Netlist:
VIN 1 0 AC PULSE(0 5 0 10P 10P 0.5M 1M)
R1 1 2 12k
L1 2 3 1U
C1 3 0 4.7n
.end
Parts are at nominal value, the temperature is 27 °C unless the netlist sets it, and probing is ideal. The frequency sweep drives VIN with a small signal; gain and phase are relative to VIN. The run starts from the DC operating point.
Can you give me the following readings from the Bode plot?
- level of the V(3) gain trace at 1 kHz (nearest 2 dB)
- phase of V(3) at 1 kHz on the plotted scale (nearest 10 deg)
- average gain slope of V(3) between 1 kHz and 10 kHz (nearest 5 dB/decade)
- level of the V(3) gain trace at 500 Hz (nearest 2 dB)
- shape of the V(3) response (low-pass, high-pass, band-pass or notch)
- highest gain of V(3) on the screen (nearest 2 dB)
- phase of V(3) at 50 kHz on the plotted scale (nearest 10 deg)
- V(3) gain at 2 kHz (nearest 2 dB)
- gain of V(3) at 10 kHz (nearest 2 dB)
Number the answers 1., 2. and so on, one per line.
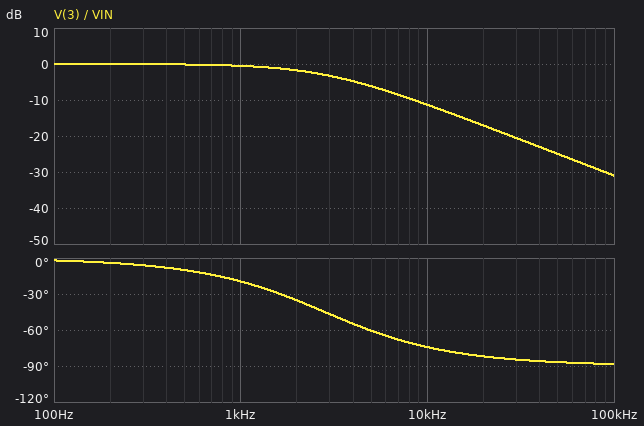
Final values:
1. 0 dB
2. -20 deg
3. -10 dB/decade
4. 0 dB
5. low-pass
6. 0 dB
7. -90 deg
8. -2 dB
9. -12 dB
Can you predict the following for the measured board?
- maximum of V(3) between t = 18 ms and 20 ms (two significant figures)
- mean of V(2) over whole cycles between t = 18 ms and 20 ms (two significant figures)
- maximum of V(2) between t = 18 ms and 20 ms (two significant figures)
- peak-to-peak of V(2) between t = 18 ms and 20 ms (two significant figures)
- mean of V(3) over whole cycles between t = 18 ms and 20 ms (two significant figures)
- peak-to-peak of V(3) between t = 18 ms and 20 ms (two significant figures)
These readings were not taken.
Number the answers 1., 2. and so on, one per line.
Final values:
1. 5.0 V
2. 2.5 V
3. 5.0 V
4. 5.0 V
5. 2.5 V
6. 5.0 V
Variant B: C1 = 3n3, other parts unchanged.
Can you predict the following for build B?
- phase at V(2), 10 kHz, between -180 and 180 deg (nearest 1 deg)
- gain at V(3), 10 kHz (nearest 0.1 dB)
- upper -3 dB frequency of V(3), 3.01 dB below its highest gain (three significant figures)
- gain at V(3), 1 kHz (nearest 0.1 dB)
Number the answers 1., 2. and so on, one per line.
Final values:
1. -68 deg
2. -8.6 dB
3. 4.02 kHz
4. -0.3 dB
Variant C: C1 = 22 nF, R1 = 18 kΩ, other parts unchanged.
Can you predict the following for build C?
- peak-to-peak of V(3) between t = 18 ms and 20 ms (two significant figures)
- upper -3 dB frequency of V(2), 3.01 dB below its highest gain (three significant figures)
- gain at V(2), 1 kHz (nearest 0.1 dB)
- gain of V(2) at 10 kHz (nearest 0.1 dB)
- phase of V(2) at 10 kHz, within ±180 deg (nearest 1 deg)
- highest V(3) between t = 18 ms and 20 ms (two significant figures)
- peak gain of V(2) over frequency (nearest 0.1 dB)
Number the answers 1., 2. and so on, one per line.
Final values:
1. 2.8 V
2. 402 Hz
3. -8.6 dB
4. -27.9 dB
5. -88 deg
6. 3.9 V
7. 0 dB
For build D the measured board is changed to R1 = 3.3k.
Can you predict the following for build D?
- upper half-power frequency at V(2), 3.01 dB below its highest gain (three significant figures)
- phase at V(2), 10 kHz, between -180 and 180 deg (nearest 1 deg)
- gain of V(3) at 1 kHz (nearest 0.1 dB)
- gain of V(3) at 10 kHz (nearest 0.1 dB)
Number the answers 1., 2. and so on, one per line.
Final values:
1. 10.3 kHz
2. -44 deg
3. 0 dB
4. -2.9 dB
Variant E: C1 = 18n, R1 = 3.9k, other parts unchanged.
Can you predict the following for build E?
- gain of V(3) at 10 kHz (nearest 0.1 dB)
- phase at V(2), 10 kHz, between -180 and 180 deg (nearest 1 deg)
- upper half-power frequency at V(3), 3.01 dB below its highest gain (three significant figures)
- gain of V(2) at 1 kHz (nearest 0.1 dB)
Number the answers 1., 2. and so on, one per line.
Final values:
1. -13.1 dB
2. -77 deg
3. 2.27 kHz
4. -0.8 dB
